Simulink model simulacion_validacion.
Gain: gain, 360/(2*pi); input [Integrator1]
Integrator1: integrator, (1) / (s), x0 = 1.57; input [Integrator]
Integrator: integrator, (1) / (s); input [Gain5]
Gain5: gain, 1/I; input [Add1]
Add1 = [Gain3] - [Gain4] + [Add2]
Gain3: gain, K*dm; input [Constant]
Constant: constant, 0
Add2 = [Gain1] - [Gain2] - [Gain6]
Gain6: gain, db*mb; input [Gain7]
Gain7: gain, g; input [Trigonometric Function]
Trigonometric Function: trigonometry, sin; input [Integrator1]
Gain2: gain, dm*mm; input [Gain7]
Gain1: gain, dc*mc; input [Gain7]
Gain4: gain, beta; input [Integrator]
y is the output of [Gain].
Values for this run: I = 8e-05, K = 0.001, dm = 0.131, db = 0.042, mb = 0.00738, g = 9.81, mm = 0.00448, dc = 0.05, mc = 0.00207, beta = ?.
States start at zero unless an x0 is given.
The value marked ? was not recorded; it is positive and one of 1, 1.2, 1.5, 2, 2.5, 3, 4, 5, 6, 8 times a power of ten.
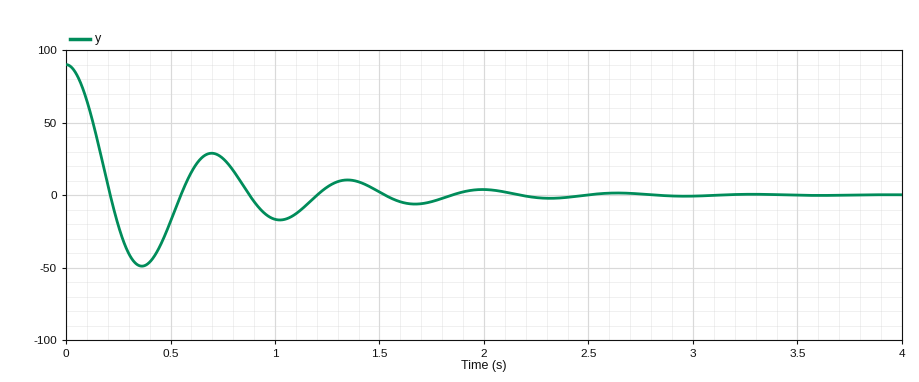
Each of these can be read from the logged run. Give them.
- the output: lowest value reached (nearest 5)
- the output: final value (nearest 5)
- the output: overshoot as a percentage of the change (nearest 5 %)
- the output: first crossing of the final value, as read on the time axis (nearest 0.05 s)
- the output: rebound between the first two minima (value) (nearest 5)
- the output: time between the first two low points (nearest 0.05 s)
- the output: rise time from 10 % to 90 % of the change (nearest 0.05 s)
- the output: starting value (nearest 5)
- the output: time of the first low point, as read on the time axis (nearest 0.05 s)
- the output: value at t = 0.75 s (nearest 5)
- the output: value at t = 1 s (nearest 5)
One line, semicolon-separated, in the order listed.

-50; 0; 55 %; 0.20 s; 30; 0.65 s; 0.15 s; 90; 0.35 s; 25; -15
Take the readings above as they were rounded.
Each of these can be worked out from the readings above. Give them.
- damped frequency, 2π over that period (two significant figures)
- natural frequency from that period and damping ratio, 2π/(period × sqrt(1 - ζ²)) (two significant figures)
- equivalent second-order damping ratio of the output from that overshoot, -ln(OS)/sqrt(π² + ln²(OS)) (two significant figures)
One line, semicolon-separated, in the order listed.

9.7 rad/s; 9.8 rad/s; 0.19
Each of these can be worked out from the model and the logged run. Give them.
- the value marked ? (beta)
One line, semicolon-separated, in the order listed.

0.00025
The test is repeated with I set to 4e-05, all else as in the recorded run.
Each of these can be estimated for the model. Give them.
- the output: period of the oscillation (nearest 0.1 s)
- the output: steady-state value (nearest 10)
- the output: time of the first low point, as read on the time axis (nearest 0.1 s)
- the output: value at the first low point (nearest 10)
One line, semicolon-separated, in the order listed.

0.5 s; 0; 0.3 s; -40
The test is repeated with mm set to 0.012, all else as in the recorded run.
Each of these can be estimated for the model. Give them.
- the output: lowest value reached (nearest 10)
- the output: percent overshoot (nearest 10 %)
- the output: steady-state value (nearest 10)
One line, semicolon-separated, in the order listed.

-60; 70 %; 0
